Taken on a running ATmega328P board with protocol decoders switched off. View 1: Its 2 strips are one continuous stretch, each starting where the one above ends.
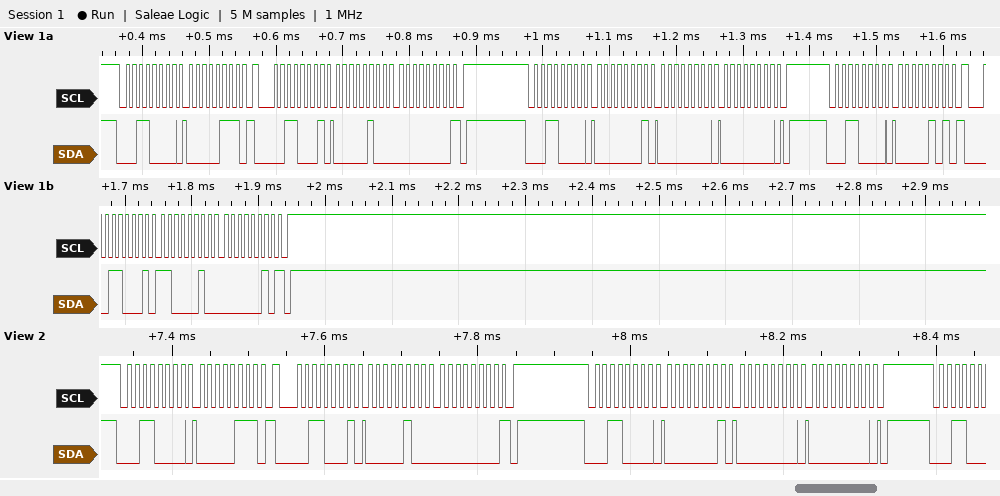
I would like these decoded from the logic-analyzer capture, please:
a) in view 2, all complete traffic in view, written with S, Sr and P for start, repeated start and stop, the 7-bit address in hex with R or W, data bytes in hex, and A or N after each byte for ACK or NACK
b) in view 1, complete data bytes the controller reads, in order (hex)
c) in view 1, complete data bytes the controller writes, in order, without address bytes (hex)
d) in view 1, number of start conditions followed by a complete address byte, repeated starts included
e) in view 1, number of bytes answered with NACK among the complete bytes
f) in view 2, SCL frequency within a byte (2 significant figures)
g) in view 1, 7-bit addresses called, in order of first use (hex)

S 18W A 07 A Sr 18R A 04 A 00 N P S 18W A 01 A 00 A 00 A P
04 00 C2 02
07 01 00 00 05
5
2
100 kHz
0x18
